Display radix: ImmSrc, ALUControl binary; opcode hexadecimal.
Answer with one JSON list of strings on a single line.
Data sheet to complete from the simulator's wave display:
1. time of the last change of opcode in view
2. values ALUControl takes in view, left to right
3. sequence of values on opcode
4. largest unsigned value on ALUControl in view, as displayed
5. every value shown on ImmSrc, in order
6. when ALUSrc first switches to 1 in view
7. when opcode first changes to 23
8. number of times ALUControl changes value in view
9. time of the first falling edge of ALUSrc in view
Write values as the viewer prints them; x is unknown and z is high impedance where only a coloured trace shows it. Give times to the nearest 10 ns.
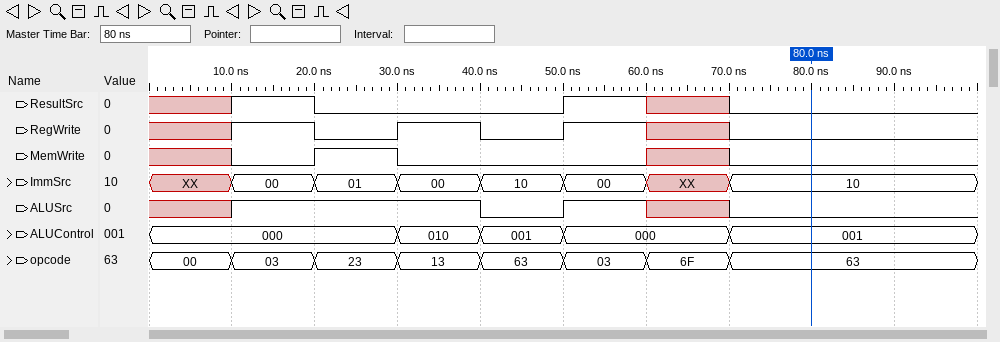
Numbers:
["70 ns", "000, 010, 001, 000, 001", "00, 03, 23, 13, 63, 03, 6F, 63", "010", "XX, 00, 01, 00, 10, 00, XX, 10", "10 ns", "20 ns", "4", "40 ns"]
